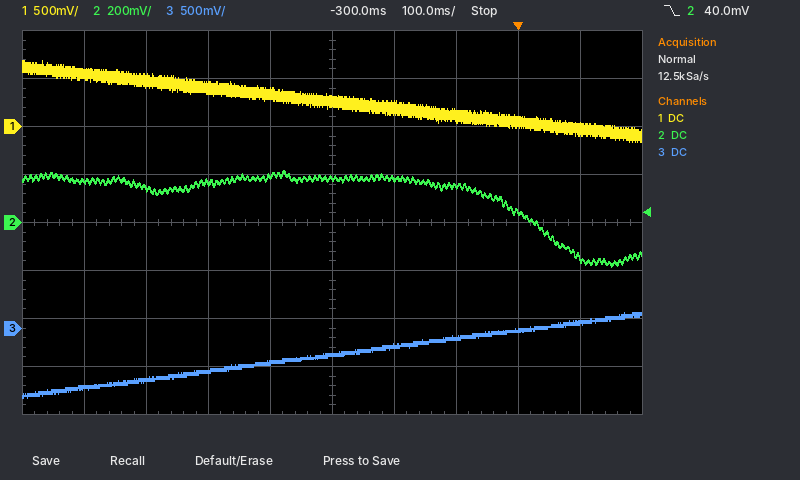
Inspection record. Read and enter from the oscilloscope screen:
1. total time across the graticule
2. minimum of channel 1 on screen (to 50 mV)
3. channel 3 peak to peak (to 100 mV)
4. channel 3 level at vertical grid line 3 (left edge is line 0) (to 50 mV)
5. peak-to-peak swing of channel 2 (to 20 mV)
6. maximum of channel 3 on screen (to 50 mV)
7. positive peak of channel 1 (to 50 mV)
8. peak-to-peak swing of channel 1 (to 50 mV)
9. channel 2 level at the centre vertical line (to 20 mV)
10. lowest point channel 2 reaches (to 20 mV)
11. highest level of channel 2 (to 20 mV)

1 s
-150 mV
900 mV
-450 mV
400 mV
150 mV
700 mV
850 mV
180 mV
-180 mV
220 mV
